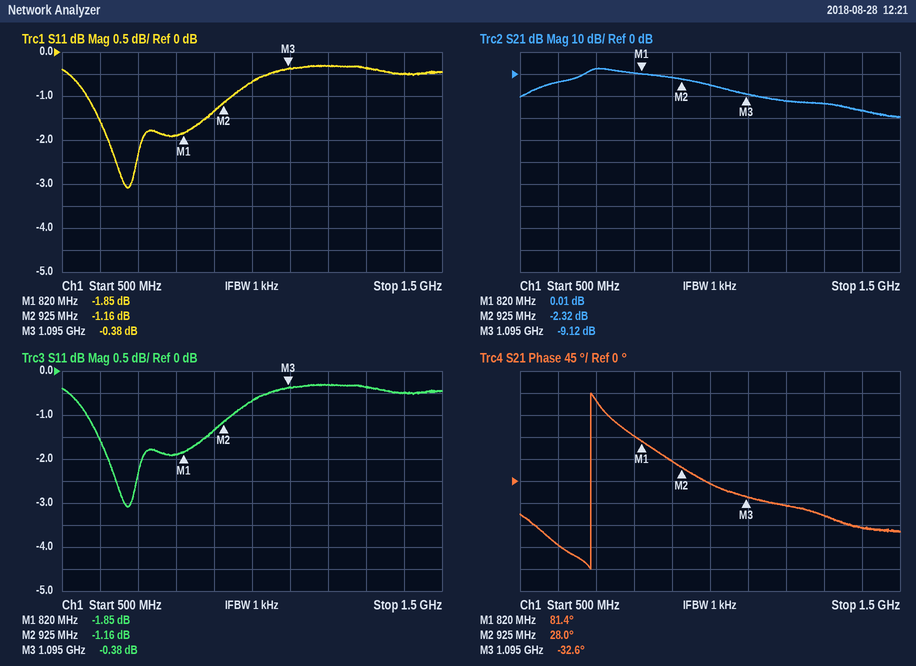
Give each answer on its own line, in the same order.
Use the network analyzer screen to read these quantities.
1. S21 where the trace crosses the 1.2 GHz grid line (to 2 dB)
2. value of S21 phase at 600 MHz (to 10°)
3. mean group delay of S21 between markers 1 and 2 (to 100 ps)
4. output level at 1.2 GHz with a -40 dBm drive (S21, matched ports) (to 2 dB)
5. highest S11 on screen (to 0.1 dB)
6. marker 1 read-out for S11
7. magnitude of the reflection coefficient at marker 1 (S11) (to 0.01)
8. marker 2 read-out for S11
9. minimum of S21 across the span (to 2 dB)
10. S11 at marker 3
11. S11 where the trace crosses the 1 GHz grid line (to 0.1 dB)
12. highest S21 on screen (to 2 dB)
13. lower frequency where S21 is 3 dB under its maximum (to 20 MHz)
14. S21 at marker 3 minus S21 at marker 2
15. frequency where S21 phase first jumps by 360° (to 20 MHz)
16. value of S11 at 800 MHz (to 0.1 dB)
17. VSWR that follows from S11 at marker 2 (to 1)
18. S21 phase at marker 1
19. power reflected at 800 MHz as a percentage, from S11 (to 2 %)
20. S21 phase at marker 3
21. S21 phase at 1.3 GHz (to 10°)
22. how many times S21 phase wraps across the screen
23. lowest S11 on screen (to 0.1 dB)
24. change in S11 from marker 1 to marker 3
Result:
-12 dB
-130°
1.4 ns
-52 dBm
-0.3 dB
-1.85 dB
0.81
-1.16 dB
-20 dB
-0.38 dB
-0.7 dB
2 dB
660 MHz
-6.80 dB
680 MHz
-1.9 dB
15
81.4°
64 %
-32.6°
-70°
1
-3.1 dB
1.47 dB
